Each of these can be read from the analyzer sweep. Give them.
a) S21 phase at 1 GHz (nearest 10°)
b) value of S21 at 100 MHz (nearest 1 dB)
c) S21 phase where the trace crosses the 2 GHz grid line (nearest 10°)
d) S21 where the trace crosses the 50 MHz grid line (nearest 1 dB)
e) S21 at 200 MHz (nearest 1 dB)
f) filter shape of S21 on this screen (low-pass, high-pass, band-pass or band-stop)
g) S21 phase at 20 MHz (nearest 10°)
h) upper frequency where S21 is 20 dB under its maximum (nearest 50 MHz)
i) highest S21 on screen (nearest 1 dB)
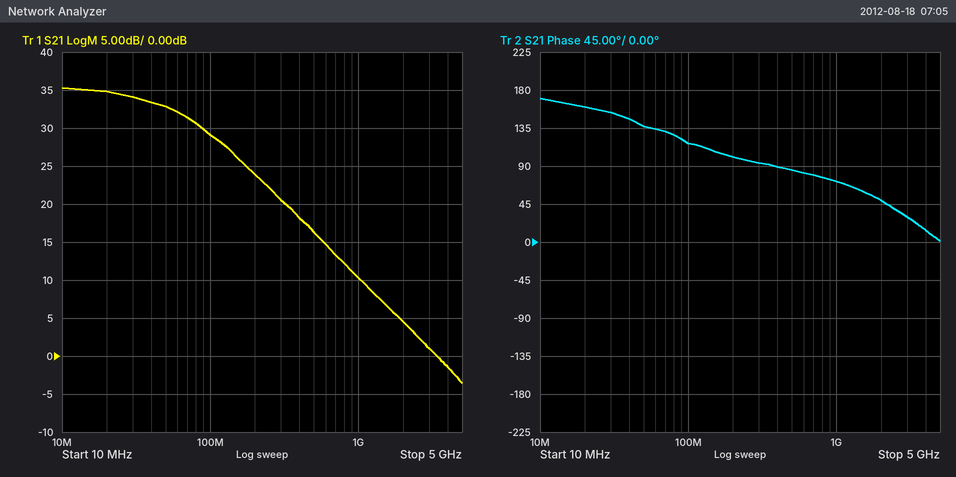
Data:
70°
29 dB
50°
33 dB
24 dB
low-pass
160°
550 MHz
35 dB
